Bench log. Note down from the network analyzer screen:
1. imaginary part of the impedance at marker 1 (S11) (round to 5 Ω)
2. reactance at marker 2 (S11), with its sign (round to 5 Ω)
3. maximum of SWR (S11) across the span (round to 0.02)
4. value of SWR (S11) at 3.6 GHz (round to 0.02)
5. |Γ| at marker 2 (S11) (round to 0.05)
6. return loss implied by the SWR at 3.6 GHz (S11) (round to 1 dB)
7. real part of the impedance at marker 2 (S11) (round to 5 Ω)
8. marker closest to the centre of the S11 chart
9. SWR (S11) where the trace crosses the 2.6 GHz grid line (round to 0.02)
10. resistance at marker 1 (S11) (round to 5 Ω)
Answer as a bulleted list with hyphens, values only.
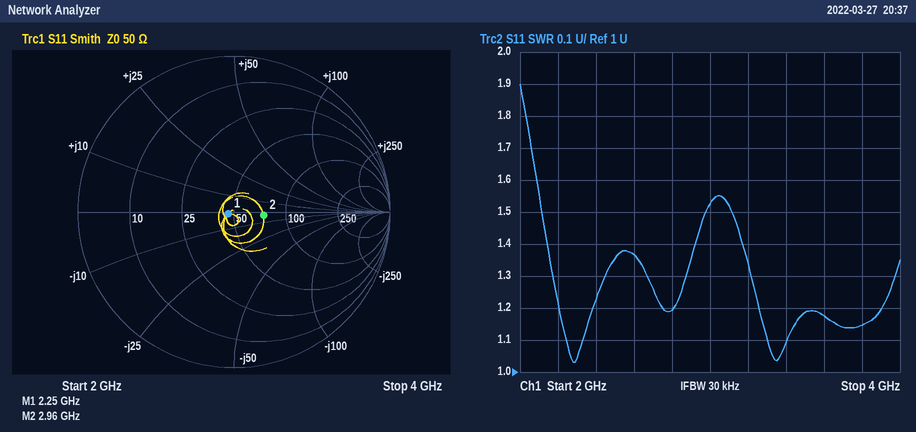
- 0 Ω
- -5 Ω
- 1.90
- 1.18
- 0.20
- 22 dB
- 75 Ω
- marker 1
- 1.36
- 45 Ω
